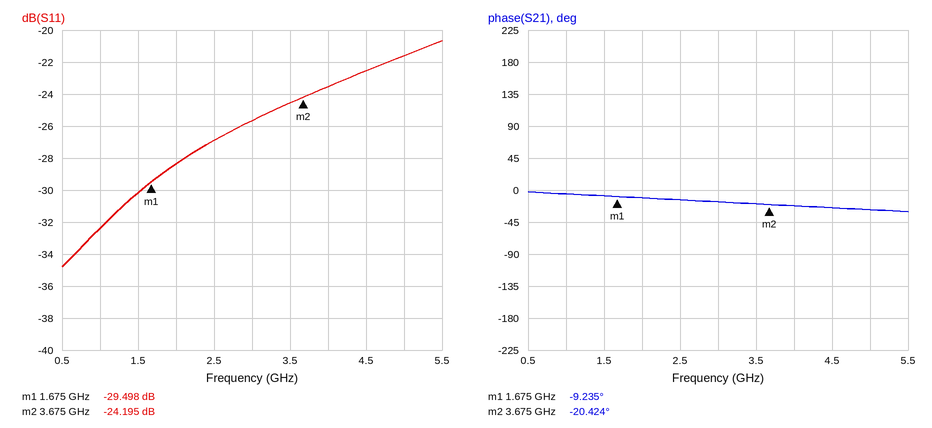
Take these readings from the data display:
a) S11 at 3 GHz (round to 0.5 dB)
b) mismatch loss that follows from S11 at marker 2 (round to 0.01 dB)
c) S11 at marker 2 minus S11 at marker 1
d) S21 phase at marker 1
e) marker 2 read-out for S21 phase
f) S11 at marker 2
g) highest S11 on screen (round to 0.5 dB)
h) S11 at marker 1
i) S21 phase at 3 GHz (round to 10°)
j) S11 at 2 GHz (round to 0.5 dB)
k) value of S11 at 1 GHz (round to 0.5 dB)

-25.5 dB
0.02 dB
5.303 dB
-9.235°
-20.424°
-24.195 dB
-20.5 dB
-29.498 dB
-20°
-28.5 dB
-32.5 dB
